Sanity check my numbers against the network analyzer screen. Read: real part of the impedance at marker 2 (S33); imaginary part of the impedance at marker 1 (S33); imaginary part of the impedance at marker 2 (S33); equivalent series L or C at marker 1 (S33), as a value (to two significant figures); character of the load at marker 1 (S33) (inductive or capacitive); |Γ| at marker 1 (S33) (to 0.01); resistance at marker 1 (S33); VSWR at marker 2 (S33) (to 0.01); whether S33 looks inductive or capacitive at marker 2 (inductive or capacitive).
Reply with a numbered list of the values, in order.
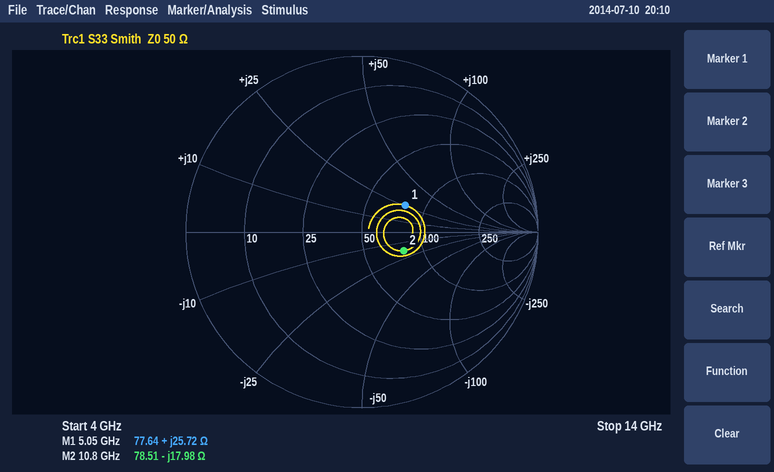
1. 78.51 Ω
2. +25.72 Ω
3. -17.98 Ω
4. 810 pH
5. inductive
6. 0.29
7. 77.64 Ω
8. 1.70
9. capacitive
